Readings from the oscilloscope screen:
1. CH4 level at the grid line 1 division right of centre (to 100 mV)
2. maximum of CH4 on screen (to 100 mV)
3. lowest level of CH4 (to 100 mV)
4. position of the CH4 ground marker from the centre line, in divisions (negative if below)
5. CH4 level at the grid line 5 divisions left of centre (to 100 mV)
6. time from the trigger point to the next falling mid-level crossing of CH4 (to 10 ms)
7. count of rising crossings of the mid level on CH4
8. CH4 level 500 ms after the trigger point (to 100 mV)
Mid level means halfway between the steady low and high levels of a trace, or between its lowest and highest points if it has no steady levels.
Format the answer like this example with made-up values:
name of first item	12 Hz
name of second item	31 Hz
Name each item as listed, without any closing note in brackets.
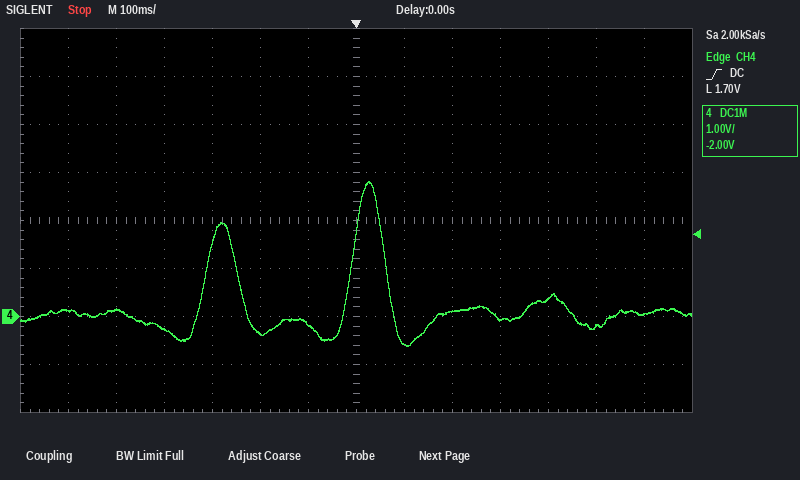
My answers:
CH4 level at the grid line 1 division right of centre	-600 mV
maximum of CH4 on screen	2.8 V
lowest level of CH4	-600 mV
position of the CH4 ground marker from the centre line, in divisions	-2.0 div
CH4 level at the grid line 5 divisions left of centre	100 mV
time from the trigger point to the next falling mid-level crossing of CH4	60 ms
count of rising crossings of the mid level on CH4	2
CH4 level 500 ms after the trigger point	-200 mV
